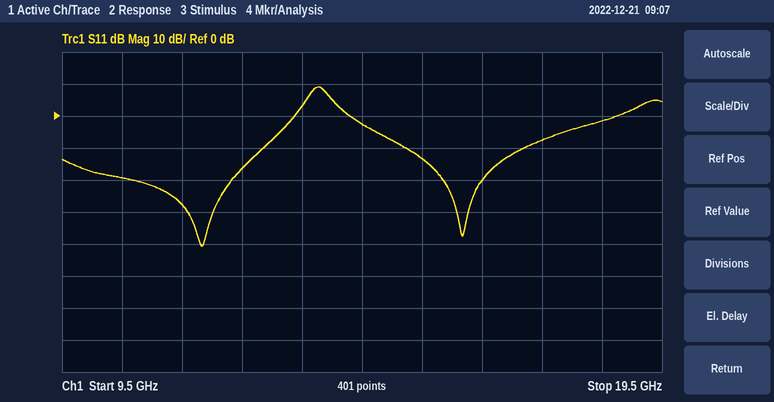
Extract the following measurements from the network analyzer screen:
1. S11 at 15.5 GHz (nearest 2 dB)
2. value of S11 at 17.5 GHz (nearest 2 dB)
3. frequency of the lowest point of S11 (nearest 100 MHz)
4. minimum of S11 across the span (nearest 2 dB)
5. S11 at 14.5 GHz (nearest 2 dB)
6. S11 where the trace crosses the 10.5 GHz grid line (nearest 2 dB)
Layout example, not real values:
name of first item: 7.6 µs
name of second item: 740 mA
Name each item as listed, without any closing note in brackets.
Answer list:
S11 at 15.5 GHz: -14 dB
value of S11 at 17.5 GHz: -8 dB
frequency of the lowest point of S11: 11.8 GHz
minimum of S11 across the span: -40 dB
S11 at 14.5 GHz: -2 dB
S11 where the trace crosses the 10.5 GHz grid line: -20 dB
